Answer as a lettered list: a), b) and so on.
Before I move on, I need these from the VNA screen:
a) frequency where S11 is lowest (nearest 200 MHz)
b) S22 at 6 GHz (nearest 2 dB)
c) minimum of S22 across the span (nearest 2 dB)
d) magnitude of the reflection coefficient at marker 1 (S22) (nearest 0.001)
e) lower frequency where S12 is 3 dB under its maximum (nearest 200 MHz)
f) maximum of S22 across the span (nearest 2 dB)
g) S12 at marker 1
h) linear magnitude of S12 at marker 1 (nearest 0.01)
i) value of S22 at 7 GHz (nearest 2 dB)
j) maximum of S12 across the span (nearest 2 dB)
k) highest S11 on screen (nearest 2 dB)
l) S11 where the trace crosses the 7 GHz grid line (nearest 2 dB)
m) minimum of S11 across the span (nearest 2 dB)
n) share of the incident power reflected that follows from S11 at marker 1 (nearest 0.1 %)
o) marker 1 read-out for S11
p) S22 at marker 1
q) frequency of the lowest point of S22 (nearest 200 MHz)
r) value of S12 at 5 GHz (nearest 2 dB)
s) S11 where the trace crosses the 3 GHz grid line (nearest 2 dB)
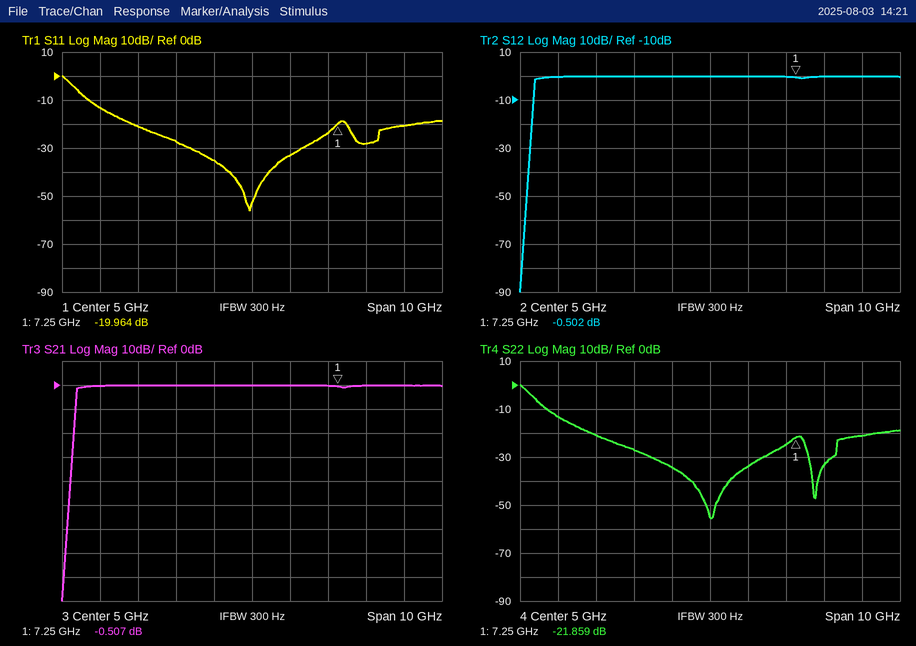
a) 5.0 GHz
b) -34 dB
c) -56 dB
d) 0.081
e) 400 MHz
f) 0 dB
g) -0.502 dB
h) 0.94
i) -24 dB
j) 0 dB
k) 0 dB
l) -24 dB
m) -56 dB
n) 1.0 %
o) -19.964 dB
p) -21.859 dB
q) 5.0 GHz
r) 0 dB
s) -28 dB
